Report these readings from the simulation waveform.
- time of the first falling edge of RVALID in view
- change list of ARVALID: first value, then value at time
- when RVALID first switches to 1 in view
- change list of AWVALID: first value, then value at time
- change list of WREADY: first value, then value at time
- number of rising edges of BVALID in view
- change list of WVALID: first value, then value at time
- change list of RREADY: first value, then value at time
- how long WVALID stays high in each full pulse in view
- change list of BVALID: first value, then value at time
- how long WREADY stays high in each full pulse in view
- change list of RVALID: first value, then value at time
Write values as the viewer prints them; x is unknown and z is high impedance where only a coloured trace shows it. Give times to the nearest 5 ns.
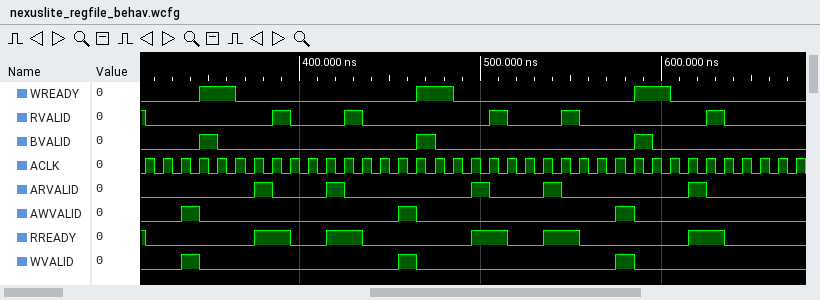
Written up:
315 ns
0, 1 at 375 ns, 0 at 385 ns, 1 at 415 ns, 0 at 425 ns, 1 at 495 ns, 0 at 505 ns, 1 at 535 ns, 0 at 545 ns, 1 at 615 ns, 0 at 625 ns
385 ns
0, 1 at 335 ns, 0 at 345 ns, 1 at 455 ns, 0 at 465 ns, 1 at 575 ns, 0 at 585 ns
0, 1 at 345 ns, 0 at 365 ns, 1 at 465 ns, 0 at 485 ns, 1 at 585 ns, 0 at 605 ns
3
0, 1 at 335 ns, 0 at 345 ns, 1 at 455 ns, 0 at 465 ns, 1 at 575 ns, 0 at 585 ns
1, 0 at 315 ns, 1 at 375 ns, 0 at 395 ns, 1 at 415 ns, 0 at 435 ns, 1 at 495 ns, 0 at 515 ns, 1 at 535 ns, 0 at 555 ns, 1 at 615 ns, 0 at 635 ns
10 ns, 10 ns, 10 ns
0, 1 at 345 ns, 0 at 355 ns, 1 at 465 ns, 0 at 475 ns, 1 at 585 ns, 0 at 595 ns
20 ns, 20 ns, 20 ns
1, 0 at 315 ns, 1 at 385 ns, 0 at 395 ns, 1 at 425 ns, 0 at 435 ns, 1 at 505 ns, 0 at 515 ns, 1 at 545 ns, 0 at 555 ns, 1 at 625 ns, 0 at 635 ns
